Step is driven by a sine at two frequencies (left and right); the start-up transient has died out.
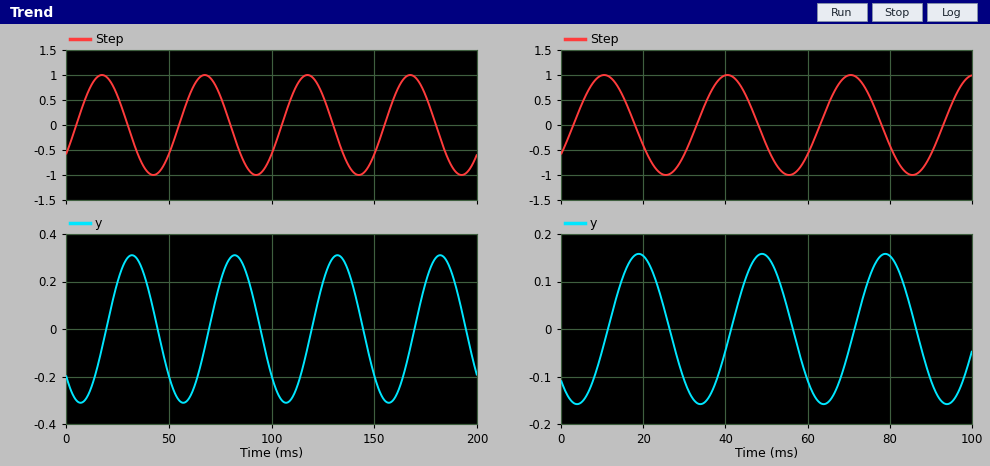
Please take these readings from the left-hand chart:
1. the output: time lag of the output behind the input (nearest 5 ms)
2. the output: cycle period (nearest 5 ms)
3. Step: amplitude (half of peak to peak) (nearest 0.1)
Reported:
15 ms
50 ms
1.0
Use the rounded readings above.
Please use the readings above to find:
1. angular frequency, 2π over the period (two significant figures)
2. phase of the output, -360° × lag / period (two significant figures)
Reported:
0.13 rad/ms
-110°
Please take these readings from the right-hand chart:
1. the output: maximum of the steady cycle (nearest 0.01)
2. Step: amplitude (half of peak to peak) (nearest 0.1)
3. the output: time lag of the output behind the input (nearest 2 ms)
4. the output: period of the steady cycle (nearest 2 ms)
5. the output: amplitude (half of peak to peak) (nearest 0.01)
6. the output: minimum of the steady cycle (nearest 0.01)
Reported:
0.16
1.0
8 ms
30 ms
0.16
-0.16
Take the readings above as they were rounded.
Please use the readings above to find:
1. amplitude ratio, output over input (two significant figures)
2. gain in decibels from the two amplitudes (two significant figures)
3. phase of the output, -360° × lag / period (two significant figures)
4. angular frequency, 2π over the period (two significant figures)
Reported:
0.16
-16 dB
-96°
0.21 rad/ms
